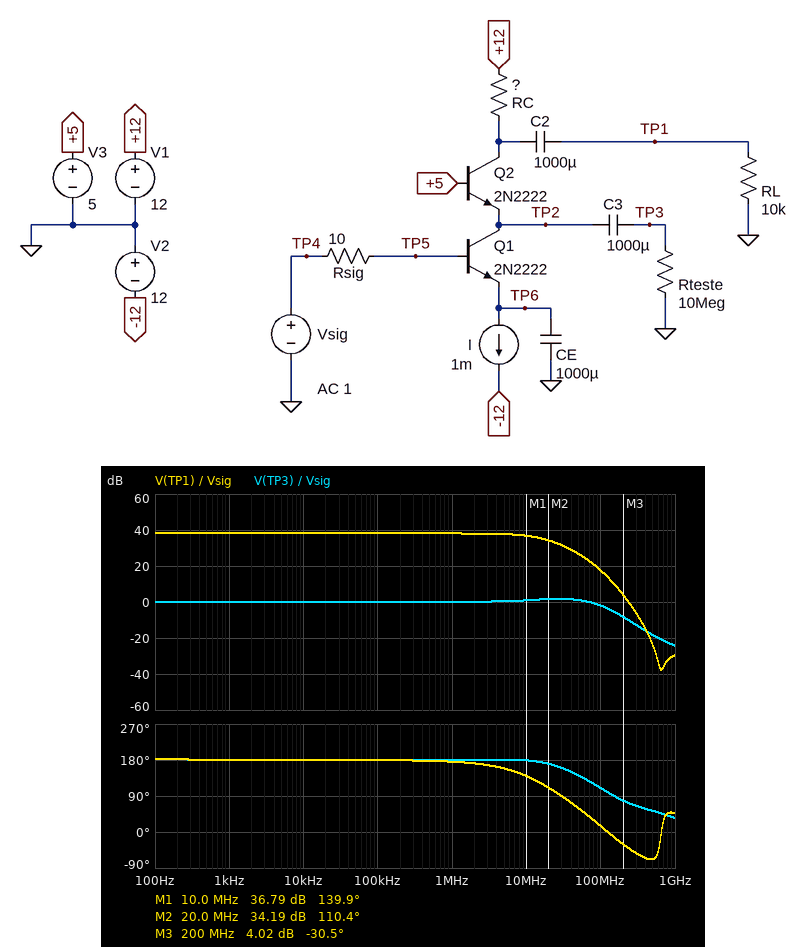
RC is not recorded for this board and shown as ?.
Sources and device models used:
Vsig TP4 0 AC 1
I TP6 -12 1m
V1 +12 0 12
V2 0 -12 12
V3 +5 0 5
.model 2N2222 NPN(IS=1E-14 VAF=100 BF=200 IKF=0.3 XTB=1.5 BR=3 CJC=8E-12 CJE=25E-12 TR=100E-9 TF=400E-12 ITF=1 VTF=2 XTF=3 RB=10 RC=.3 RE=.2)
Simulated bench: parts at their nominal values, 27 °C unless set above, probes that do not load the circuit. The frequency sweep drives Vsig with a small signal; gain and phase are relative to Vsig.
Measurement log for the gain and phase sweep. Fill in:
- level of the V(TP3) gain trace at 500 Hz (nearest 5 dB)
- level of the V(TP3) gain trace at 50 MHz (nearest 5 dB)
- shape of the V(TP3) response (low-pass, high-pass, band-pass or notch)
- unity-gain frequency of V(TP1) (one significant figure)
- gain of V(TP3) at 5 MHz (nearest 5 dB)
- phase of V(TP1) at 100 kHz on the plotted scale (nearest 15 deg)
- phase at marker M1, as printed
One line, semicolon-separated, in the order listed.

0 dB; 0 dB; low-pass; 200 MHz; 0 dB; 180 deg; 139.9 deg
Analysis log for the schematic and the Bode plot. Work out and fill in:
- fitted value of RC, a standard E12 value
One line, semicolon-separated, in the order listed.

2.7 kΩ
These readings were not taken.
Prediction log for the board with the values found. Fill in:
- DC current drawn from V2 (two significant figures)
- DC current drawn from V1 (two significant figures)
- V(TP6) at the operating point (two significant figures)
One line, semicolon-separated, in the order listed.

1.0 mA; 990 µA; -650 mV
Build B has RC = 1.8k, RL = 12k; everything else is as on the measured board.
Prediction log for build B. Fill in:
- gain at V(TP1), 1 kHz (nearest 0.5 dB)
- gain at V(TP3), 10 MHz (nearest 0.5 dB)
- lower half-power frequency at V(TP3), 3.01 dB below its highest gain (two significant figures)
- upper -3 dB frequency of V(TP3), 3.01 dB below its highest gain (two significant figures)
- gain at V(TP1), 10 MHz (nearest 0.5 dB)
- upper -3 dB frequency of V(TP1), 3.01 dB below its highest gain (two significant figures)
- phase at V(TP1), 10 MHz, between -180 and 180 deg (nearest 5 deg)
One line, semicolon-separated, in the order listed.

35.5 dB; 0.5 dB; 8.7 Hz; 94 MHz; 34.5 dB; 23 MHz; 150 deg
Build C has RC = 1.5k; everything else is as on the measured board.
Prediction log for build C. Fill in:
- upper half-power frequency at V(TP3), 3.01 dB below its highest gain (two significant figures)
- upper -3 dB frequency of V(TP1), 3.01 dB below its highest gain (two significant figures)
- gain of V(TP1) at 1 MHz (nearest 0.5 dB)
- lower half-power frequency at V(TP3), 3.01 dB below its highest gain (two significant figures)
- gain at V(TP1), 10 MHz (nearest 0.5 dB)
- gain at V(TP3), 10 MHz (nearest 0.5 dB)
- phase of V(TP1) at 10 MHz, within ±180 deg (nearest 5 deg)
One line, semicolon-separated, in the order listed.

97 MHz; 27 MHz; 34.0 dB; 8.2 Hz; 33.5 dB; 0.5 dB; 150 deg
